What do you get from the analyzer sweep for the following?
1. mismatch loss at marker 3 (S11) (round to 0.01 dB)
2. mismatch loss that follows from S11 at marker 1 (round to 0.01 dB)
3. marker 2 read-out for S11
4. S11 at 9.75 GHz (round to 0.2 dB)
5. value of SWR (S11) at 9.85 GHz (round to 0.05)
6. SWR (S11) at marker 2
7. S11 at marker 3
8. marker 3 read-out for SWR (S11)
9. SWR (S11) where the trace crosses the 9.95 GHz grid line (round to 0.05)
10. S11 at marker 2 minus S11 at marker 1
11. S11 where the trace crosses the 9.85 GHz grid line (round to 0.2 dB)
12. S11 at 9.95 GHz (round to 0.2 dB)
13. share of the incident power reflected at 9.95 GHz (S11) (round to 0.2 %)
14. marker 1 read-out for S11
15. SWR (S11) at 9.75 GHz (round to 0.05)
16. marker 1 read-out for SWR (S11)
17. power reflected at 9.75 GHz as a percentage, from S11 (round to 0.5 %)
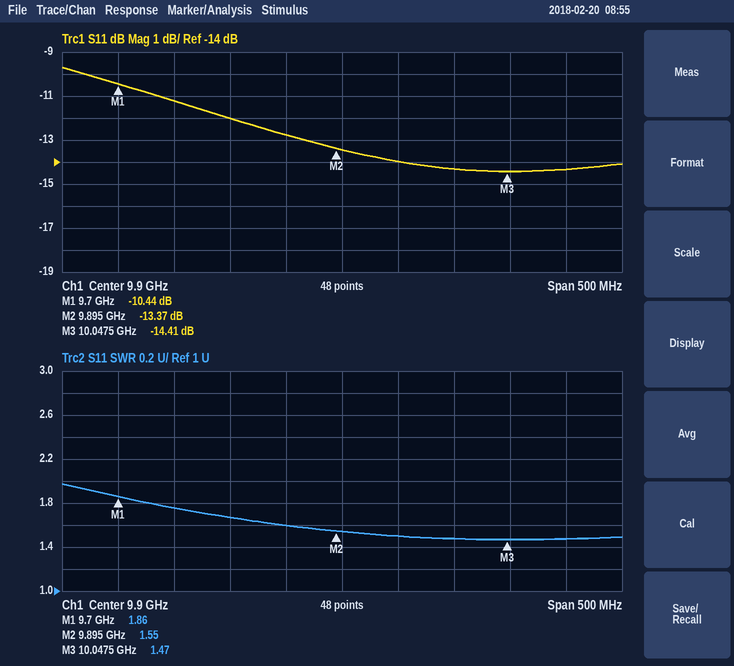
0.16 dB
0.41 dB
-13.37 dB
-11.2 dB
1.60
1.55
-14.41 dB
1.47
1.50
-2.93 dB
-12.8 dB
-14.0 dB
4.0 %
-10.44 dB
1.75
1.86
7.5 %
